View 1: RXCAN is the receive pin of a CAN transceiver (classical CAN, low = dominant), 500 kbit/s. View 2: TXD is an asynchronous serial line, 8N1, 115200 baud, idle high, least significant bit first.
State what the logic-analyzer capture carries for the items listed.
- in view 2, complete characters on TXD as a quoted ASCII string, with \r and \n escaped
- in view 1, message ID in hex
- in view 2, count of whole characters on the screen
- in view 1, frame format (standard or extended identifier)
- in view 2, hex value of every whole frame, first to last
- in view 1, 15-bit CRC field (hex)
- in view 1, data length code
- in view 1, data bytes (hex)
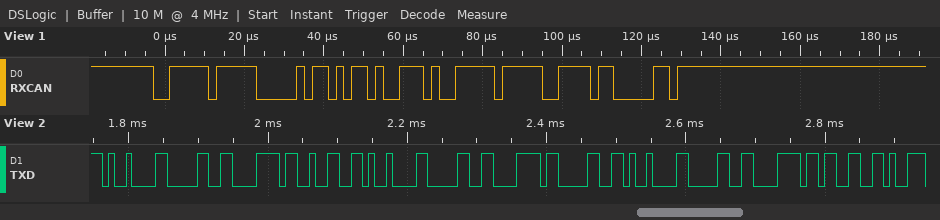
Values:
"\t0x2\t0x0\t0x3"
0x3FF
12
standard
09 30 78 32 09 30 78 30 09 30 78 33
0x6F60
3
5A 74 FF
